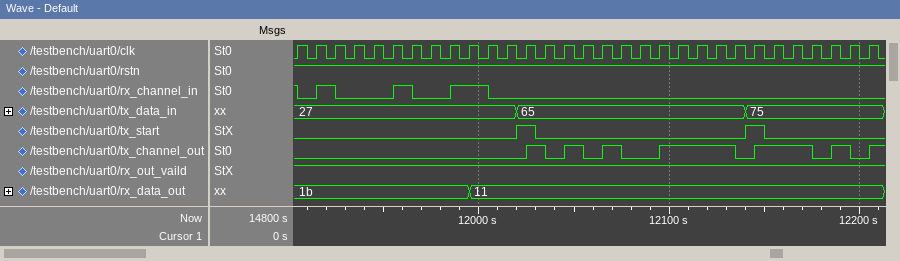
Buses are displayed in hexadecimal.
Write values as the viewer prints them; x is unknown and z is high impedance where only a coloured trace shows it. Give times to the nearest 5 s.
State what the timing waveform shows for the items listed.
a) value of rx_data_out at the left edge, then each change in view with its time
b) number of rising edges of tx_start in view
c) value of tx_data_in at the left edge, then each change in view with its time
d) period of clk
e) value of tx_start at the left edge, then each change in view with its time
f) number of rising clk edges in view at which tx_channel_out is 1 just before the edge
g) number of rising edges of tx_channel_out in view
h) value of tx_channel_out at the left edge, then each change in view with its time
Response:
1b, 11 at 11995 s
2
27, 65 at 12020 s, 75 at 12140 s
10 s
0, 1 at 12020 s, 0 at 12030 s, 1 at 12140 s, 0 at 12150 s
11
7
0, 1 at 12025 s, 0 at 12035 s, 1 at 12045 s, 0 at 12055 s, 1 at 12065 s, 0 at 12075 s, 1 at 12095 s, 0 at 12135 s, 1 at 12145 s, 0 at 12175 s, 1 at 12185 s, 0 at 12195 s, 1 at 12205 s
